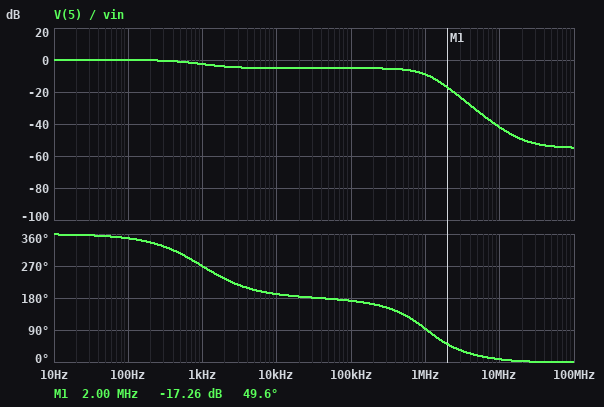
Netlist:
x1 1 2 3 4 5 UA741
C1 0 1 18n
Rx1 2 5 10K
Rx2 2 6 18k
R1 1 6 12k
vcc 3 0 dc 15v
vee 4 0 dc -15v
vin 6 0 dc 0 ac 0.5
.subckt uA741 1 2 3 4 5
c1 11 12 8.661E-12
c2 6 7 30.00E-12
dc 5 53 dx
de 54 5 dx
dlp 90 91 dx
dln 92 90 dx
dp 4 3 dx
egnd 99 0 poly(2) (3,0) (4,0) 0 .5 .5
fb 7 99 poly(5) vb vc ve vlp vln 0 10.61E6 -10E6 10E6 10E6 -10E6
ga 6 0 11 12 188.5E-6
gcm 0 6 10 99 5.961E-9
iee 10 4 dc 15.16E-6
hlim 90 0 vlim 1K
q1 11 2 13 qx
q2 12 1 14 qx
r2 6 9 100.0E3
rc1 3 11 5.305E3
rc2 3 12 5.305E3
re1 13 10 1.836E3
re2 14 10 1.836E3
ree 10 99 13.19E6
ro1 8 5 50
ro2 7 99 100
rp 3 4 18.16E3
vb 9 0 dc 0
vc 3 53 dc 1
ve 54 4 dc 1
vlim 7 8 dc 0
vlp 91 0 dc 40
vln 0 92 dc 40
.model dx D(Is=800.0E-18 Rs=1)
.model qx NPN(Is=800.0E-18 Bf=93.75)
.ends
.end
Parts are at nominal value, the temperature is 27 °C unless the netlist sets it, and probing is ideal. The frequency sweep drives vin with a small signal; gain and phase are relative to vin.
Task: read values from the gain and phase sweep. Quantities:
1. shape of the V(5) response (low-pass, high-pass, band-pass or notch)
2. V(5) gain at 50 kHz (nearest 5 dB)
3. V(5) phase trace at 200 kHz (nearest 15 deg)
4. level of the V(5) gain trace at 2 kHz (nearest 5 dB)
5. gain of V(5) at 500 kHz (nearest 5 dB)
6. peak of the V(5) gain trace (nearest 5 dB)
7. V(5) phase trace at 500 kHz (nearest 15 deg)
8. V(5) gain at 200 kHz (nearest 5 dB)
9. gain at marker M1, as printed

low-pass
-5 dB
165 deg
-5 dB
-5 dB
0 dB
135 deg
-5 dB
-17.26 dB
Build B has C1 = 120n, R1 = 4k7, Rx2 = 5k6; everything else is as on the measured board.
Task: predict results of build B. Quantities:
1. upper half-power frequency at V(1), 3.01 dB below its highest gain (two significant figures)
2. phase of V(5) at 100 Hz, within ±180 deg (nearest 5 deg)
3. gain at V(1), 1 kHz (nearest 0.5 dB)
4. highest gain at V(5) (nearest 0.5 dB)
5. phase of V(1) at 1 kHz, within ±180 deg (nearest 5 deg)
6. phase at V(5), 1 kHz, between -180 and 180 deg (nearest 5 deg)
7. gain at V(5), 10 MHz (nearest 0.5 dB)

280 Hz
-50 deg
-11.5 dB
5.0 dB
-75 deg
-155 deg
-37.0 dB
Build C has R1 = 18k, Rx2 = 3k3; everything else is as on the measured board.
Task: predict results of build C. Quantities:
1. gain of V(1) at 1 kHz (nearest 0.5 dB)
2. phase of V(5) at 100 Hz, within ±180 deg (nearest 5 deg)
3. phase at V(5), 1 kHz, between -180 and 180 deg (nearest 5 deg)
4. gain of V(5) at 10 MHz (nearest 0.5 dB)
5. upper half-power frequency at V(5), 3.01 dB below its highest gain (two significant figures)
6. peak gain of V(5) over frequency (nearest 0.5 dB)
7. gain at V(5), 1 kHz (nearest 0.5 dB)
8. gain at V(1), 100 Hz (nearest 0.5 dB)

-7.0 dB
-45 deg
-145 deg
-35.5 dB
290 kHz
9.5 dB
9.0 dB
0 dB
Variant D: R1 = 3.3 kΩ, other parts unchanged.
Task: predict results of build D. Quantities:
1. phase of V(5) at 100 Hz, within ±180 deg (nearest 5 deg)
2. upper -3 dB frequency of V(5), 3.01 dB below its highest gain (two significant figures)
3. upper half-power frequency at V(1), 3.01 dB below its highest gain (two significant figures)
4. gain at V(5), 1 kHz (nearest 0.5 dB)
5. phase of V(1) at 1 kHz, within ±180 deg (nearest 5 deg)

-5 deg
4.3 kHz
2.7 kHz
-0.5 dB
-20 deg
